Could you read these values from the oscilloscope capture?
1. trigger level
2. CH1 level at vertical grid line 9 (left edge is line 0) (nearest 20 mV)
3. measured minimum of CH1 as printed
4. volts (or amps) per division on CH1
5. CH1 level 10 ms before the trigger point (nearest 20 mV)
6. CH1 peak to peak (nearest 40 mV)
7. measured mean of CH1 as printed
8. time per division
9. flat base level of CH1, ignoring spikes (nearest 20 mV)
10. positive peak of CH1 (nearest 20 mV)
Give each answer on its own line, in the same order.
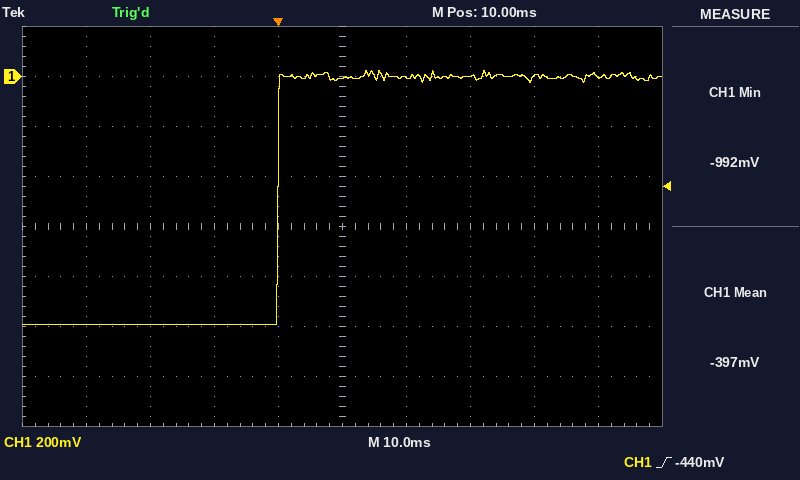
-440 mV
0 mV
-992 mV
200 mV
-1.00 V
1.00 V
-397 mV
10 ms
-1.00 V
20 mV
